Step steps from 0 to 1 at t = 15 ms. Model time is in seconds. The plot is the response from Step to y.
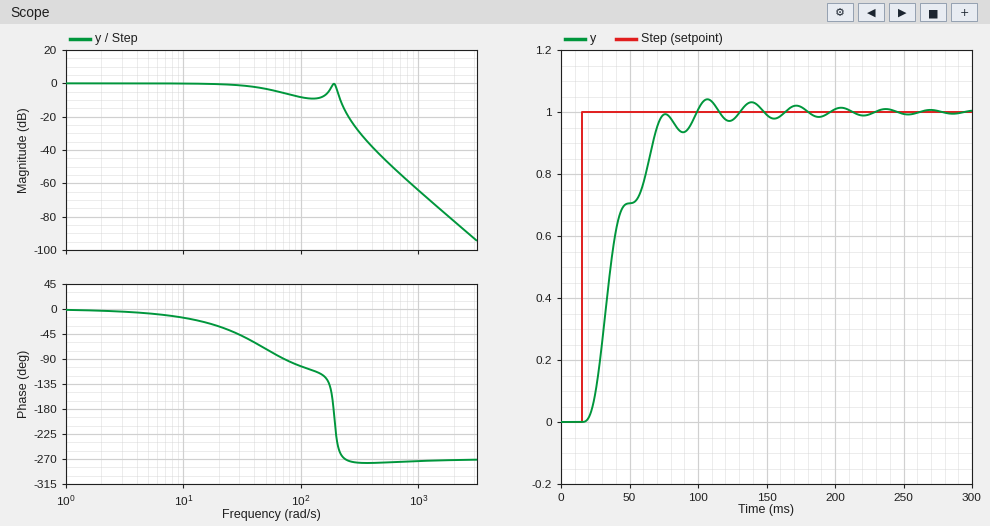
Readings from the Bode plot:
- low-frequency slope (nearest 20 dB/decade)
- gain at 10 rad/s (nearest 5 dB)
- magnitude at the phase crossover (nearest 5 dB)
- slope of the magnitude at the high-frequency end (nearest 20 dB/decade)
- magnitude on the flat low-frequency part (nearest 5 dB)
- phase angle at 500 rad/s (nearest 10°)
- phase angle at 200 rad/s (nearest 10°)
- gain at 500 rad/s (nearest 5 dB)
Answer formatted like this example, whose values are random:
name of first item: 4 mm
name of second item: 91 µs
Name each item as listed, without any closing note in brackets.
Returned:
low-frequency slope: 0 dB/decade
gain at 10 rad/s: 0 dB
magnitude at the phase crossover: 0 dB
slope of the magnitude at the high-frequency end: -60 dB/decade
magnitude on the flat low-frequency part: 0 dB
phase angle at 500 rad/s: -280°
phase angle at 200 rad/s: -230°
gain at 500 rad/s: -45 dB
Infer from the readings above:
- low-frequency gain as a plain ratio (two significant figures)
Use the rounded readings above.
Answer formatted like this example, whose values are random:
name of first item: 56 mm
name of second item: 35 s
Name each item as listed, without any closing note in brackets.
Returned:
low-frequency gain as a plain ratio: 1.0
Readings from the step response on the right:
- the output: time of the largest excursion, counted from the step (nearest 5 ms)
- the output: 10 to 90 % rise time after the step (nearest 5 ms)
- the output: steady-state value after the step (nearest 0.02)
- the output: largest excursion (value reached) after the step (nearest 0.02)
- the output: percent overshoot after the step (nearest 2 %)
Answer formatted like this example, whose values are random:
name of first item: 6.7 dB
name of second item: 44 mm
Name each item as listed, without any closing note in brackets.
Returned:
the output: time of the largest excursion, counted from the step: 90 ms
the output: 10 to 90 % rise time after the step: 40 ms
the output: steady-state value after the step: 1.00
the output: largest excursion (value reached) after the step: 1.04
the output: percent overshoot after the step: 4 %
